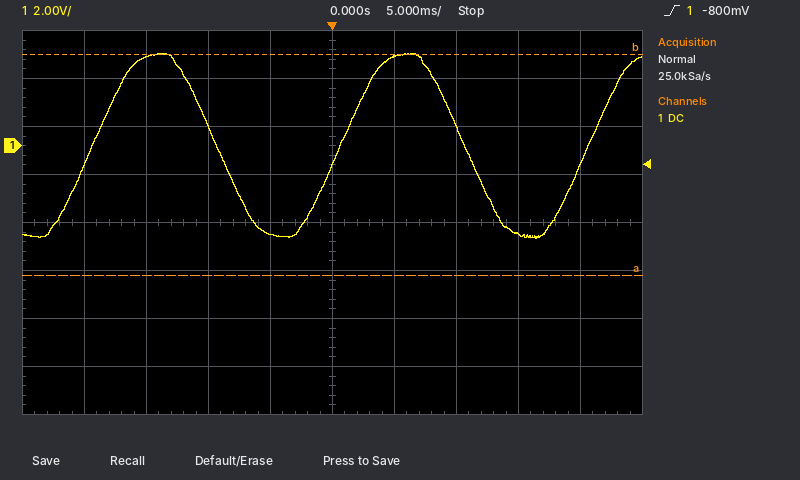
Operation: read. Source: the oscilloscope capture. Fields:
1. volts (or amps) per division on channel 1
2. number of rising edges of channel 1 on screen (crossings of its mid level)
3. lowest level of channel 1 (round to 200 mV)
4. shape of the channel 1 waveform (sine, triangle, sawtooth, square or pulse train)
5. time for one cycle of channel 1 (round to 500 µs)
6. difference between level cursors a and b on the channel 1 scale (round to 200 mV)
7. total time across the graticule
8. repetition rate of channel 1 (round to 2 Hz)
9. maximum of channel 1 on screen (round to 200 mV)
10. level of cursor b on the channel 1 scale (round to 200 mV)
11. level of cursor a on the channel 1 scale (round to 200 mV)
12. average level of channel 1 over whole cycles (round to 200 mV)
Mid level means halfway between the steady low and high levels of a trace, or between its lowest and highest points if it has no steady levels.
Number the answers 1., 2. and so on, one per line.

1. 2 V
2. 3
3. -3.8 V
4. sine
5. 20.0 ms
6. 9.2 V
7. 50 ms
8. 50 Hz
9. 3.8 V
10. 3.8 V
11. -5.4 V
12. 0.0 V
